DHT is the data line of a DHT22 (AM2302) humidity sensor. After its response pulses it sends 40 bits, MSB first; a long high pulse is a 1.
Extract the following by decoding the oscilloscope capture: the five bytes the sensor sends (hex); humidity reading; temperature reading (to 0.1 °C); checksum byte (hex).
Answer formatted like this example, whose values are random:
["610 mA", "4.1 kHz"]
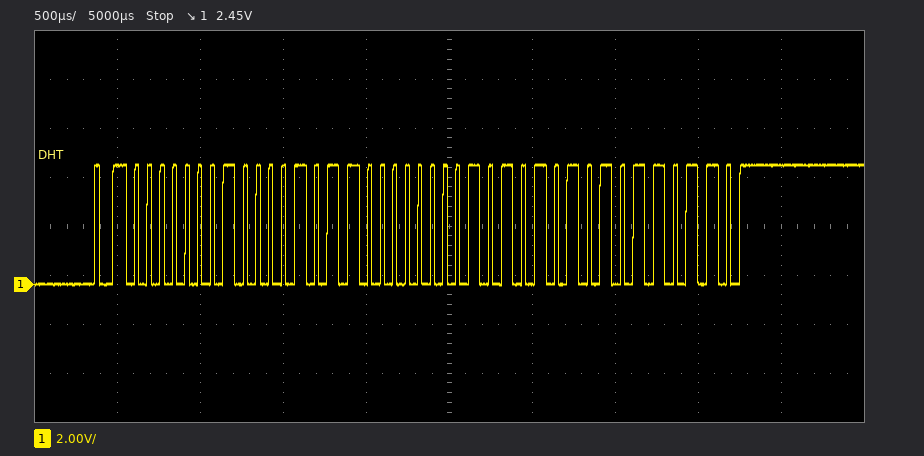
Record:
["01 0B 00 AA B6", "26.7 %", "17.0 °C", "0xB6"]
